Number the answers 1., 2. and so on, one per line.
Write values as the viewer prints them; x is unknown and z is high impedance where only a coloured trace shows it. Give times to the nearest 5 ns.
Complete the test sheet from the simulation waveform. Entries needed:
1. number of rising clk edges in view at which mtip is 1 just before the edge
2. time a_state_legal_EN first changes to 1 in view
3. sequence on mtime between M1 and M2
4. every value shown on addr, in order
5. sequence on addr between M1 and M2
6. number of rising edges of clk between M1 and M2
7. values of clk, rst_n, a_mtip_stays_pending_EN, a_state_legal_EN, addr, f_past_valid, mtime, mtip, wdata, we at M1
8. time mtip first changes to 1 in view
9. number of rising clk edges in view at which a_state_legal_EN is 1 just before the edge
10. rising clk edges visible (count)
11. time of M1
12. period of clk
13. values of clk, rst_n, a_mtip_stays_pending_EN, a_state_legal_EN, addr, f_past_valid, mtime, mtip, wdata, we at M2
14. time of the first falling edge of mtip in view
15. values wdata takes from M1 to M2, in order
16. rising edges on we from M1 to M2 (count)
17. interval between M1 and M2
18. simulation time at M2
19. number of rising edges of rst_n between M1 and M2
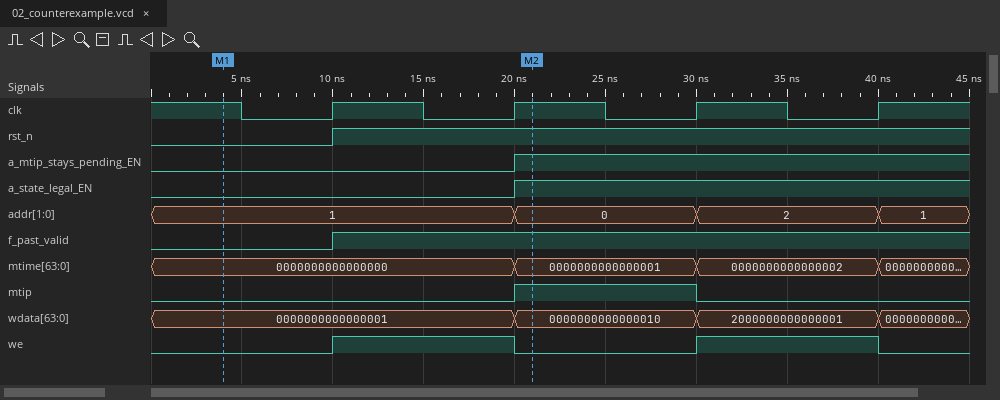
1. 1
2. 20 ns
3. 0000000000000000, 0000000000000001
4. 1, 0, 2, 1
5. 1, 0
6. 2
7. clk=1, rst_n=0, a_mtip_stays_pending_EN=0, a_state_legal_EN=0, addr=1, f_past_valid=0, mtime=0000000000000000, mtip=0, wdata=0000000000000001, we=0
8. 20 ns
9. 2
10. 4
11. 5 ns
12. 10 ns
13. clk=1, rst_n=1, a_mtip_stays_pending_EN=1, a_state_legal_EN=1, addr=0, f_past_valid=1, mtime=0000000000000001, mtip=1, wdata=0000000000000010, we=0
14. 30 ns
15. 0000000000000001, 0000000000000010
16. 1
17. 15 ns
18. 20 ns
19. 1
